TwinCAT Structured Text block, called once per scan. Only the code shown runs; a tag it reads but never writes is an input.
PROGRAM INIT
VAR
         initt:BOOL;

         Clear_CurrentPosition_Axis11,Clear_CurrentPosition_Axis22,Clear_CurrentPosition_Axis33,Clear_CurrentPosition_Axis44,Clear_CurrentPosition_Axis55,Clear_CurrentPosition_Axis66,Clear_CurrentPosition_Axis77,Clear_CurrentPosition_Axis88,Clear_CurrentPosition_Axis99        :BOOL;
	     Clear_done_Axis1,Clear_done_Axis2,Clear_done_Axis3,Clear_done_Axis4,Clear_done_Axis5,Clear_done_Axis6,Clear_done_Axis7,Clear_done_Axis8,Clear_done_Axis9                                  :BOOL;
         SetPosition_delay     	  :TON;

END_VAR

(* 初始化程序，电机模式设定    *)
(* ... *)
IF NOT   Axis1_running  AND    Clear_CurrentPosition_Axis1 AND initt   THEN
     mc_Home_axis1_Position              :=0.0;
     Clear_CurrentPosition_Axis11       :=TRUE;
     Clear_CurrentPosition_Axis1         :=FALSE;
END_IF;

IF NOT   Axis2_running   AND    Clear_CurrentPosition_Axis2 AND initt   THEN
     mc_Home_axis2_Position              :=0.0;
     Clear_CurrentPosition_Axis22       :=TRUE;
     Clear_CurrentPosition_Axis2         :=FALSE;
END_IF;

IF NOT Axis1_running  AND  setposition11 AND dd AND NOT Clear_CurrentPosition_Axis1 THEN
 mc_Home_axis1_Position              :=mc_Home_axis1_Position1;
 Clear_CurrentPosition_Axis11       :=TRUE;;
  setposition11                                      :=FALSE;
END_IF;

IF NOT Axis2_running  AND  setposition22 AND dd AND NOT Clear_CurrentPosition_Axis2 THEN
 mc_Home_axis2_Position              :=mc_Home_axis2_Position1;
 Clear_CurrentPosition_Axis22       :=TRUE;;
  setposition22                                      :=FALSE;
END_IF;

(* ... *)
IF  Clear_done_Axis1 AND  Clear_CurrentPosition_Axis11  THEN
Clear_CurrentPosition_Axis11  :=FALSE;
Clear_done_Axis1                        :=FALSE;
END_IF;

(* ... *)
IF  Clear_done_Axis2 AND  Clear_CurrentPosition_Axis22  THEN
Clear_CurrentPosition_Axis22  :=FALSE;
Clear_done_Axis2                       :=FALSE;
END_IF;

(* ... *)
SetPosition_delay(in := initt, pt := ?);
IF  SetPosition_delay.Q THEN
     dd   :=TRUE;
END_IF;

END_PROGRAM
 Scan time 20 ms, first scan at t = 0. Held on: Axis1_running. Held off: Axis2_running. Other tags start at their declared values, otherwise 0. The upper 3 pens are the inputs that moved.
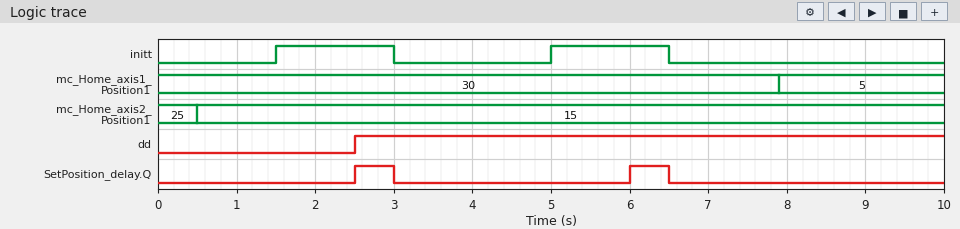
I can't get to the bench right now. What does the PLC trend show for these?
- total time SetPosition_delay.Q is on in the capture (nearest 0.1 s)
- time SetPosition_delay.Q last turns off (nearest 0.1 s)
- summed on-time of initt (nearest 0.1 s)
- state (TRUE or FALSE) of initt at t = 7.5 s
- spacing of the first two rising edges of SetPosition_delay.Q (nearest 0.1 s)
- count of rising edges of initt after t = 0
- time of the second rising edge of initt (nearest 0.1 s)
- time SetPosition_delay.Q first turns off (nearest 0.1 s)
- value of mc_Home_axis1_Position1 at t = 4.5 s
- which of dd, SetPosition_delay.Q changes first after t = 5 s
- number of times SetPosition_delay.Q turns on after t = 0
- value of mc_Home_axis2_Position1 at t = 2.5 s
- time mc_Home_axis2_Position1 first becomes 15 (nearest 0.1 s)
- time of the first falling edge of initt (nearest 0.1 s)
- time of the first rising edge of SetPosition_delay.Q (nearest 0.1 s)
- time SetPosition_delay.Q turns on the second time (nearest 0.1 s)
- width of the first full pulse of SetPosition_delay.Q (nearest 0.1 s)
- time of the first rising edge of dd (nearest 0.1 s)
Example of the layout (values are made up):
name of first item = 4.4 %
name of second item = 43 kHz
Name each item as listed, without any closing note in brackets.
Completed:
total time SetPosition_delay.Q is on in the capture = 1.0 s
time SetPosition_delay.Q last turns off = 6.5 s
summed on-time of initt = 3.0 s
state (TRUE or FALSE) of initt at t = 7.5 s = FALSE
spacing of the first two rising edges of SetPosition_delay.Q = 3.5 s
count of rising edges of initt after t = 0 = 2
time of the second rising edge of initt = 5.0 s
time SetPosition_delay.Q first turns off = 3.0 s
value of mc_Home_axis1_Position1 at t = 4.5 s = 30
which of dd, SetPosition_delay.Q changes first after t = 5 s = SetPosition_delay.Q
number of times SetPosition_delay.Q turns on after t = 0 = 2
value of mc_Home_axis2_Position1 at t = 2.5 s = 15
time mc_Home_axis2_Position1 first becomes 15 = 0.5 s
time of the first falling edge of initt = 3.0 s
time of the first rising edge of SetPosition_delay.Q = 2.5 s
time SetPosition_delay.Q turns on the second time = 6.0 s
width of the first full pulse of SetPosition_delay.Q = 0.5 s
time of the first rising edge of dd = 2.5 s
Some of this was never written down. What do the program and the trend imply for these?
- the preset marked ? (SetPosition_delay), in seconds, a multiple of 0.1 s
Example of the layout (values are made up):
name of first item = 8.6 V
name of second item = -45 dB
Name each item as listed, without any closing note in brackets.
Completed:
the preset marked ? (SetPosition_delay), in seconds, a multiple of 0.1 s = 1.0 s
